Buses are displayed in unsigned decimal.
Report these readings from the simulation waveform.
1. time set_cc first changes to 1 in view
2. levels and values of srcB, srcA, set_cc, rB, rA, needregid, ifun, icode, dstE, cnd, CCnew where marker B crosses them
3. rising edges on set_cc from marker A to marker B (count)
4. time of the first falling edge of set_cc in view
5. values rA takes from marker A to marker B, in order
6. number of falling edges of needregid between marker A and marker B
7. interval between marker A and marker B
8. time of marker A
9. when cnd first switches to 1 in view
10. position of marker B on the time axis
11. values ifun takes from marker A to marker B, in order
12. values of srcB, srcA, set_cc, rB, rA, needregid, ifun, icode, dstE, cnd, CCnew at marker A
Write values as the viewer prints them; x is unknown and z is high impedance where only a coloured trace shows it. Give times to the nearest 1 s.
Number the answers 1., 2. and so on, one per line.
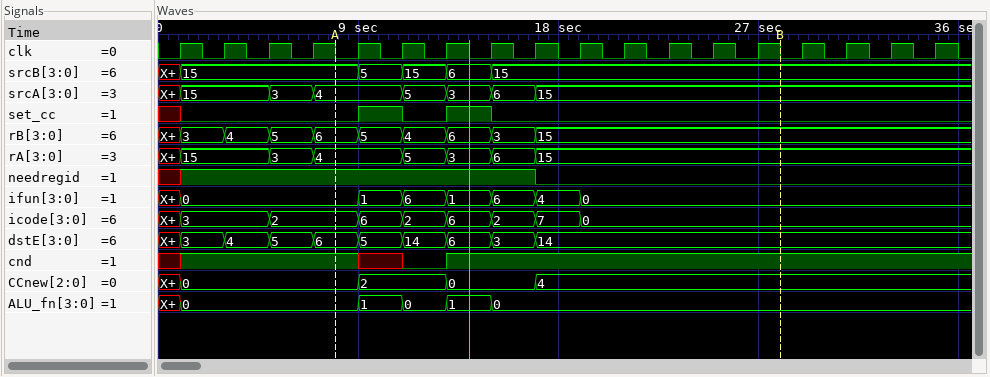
1. 9 s
2. srcB=15, srcA=15, set_cc=0, rB=15, rA=15, needregid=0, ifun=0, icode=0, dstE=14, cnd=1, CCnew=4
3. 2
4. 11 s
5. 4, 5, 3, 6, 15
6. 1
7. 20 s
8. 8 s
9. 1 s
10. 28 s
11. 0, 1, 6, 1, 6, 4, 0
12. srcB=15, srcA=4, set_cc=0, rB=6, rA=4, needregid=1, ifun=0, icode=2, dstE=6, cnd=1, CCnew=0
